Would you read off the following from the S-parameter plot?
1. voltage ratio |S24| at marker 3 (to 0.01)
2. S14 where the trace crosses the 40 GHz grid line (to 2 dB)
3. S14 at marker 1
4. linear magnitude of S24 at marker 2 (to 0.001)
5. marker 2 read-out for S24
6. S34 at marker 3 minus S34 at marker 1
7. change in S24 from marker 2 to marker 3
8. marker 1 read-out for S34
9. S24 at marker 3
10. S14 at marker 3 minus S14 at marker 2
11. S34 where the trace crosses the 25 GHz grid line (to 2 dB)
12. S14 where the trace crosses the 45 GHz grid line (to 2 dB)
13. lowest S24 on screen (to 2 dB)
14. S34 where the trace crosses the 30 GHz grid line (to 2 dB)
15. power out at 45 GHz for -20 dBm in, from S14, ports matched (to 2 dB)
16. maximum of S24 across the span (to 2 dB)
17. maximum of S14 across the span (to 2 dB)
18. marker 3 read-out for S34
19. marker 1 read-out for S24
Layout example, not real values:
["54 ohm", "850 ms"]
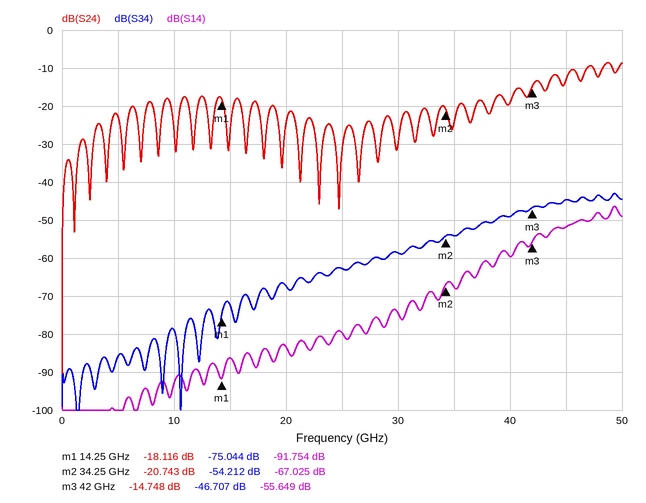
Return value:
["0.18", "-60 dB", "-91.754 dB", "0.092", "-20.743 dB", "28.337 dB", "5.995 dB", "-75.044 dB", "-14.748 dB", "11.376 dB", "-62 dB", "-52 dB", "-90 dB", "-58 dB", "-72 dBm", "-8 dB", "-46 dB", "-46.707 dB", "-18.116 dB"]
